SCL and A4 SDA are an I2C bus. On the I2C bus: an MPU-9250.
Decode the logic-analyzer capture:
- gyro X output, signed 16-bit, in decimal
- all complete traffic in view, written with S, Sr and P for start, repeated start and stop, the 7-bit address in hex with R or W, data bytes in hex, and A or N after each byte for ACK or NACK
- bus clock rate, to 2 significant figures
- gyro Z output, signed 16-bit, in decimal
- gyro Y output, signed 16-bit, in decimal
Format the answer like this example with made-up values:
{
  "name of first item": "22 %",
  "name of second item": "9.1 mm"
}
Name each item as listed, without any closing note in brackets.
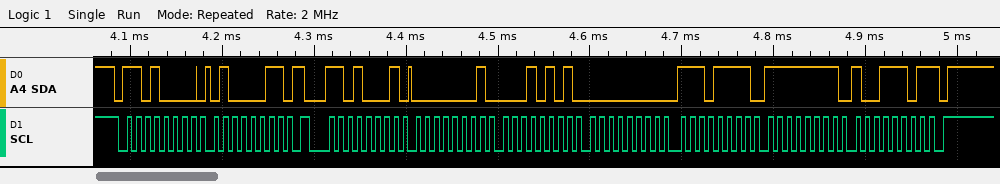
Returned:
{
  "gyro X output, signed 16-bit, in decimal": "277",
  "all complete traffic in view, written with S, Sr and P for start, repeated start and stop, the 7-bit address in hex with R or W, data bytes in hex, and A or N after each byte for ACK or NACK": "S 68W A 43 A Sr 68R A 01 A 15 A 00 A EF A FF A 9D N P",
  "bus clock rate, to 2 significant figures": "100 kHz",
  "gyro Z output, signed 16-bit, in decimal": "-99",
  "gyro Y output, signed 16-bit, in decimal": "239"
}
